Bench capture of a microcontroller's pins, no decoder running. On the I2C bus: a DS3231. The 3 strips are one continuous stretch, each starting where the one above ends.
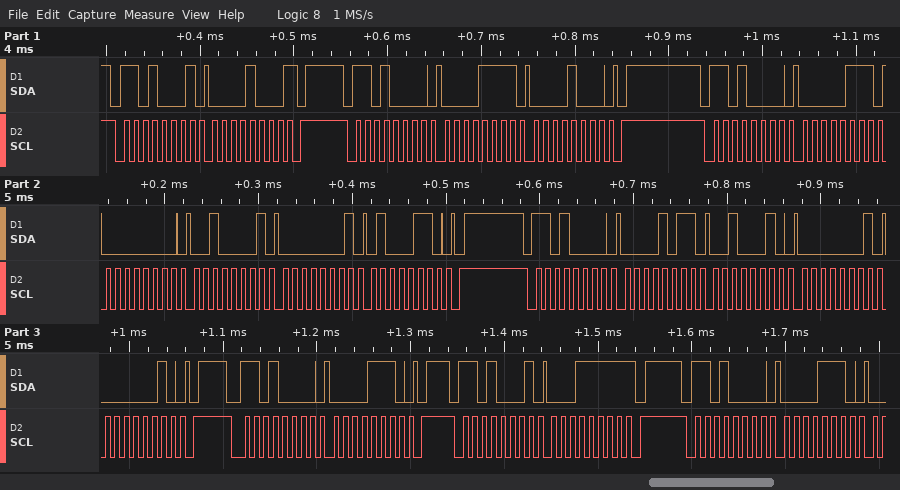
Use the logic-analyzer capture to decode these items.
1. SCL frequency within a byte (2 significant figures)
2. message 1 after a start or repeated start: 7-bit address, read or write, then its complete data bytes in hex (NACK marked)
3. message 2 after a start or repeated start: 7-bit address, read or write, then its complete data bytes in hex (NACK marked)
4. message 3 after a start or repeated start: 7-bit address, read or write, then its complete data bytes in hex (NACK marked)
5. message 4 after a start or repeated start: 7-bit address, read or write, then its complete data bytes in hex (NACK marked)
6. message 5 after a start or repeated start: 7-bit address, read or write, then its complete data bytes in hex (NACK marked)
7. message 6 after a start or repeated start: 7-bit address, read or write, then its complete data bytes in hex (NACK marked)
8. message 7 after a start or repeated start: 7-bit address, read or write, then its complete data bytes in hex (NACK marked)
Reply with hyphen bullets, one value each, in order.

- 100 kHz
- 0x68 read: 08 NACK
- 0x68 write: 0F 08
- 0x68 write: 07 00 21 01 46
- 0x68 write: 0B 22 01 02
- 0x68 write: 0E
- 0x68 read: 1F NACK
- 0x68 write: 0E
